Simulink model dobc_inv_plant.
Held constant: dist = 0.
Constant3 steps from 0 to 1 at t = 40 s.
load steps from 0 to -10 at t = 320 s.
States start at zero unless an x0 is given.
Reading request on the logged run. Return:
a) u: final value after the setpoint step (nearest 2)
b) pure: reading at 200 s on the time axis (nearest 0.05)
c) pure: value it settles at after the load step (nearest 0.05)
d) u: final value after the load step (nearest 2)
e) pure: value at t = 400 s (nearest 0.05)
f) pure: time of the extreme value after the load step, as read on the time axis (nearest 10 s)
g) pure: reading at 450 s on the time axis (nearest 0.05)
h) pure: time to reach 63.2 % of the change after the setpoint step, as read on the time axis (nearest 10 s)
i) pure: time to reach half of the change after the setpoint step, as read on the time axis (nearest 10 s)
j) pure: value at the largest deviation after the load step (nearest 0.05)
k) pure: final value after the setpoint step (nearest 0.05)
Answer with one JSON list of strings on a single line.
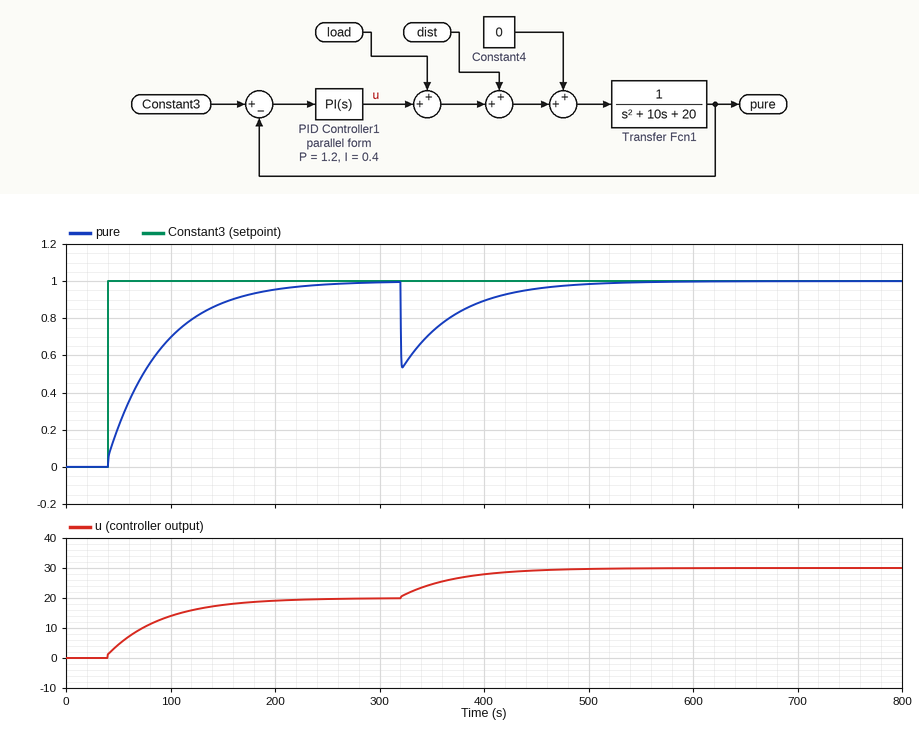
["20", "0.95", "1.00", "30", "0.90", "320 s", "0.95", "90 s", "70 s", "0.55", "1.00"]
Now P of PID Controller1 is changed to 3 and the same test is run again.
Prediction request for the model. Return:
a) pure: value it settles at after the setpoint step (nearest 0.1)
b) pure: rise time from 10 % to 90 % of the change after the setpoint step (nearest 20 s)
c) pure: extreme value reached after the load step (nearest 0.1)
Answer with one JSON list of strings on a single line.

["1.0", "120 s", "0.6"]
